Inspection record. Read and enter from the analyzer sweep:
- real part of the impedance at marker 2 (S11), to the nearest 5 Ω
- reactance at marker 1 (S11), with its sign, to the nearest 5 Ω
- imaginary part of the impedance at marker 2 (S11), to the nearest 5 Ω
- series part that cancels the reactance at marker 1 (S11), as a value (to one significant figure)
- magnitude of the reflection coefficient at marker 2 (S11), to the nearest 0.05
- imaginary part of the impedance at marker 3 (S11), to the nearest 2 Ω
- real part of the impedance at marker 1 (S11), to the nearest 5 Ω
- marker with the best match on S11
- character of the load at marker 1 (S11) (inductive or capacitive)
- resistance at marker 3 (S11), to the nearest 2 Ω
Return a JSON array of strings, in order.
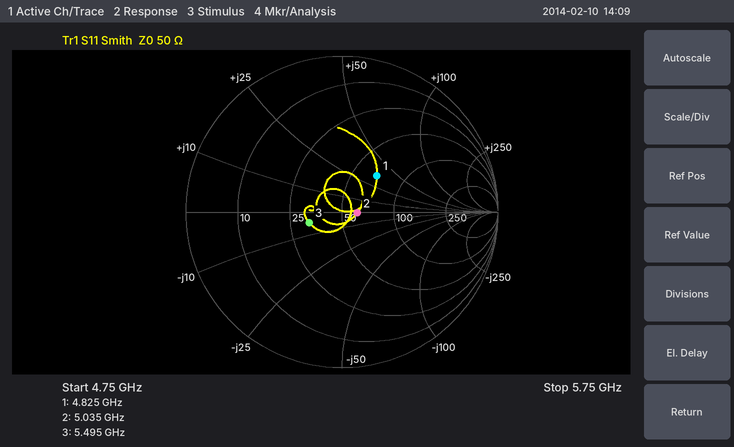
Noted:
["60 Ω", "+35 Ω", "0 Ω", "900 fF", "0.10", "-4 Ω", "70 Ω", "marker 2", "inductive", "32 Ω"]
